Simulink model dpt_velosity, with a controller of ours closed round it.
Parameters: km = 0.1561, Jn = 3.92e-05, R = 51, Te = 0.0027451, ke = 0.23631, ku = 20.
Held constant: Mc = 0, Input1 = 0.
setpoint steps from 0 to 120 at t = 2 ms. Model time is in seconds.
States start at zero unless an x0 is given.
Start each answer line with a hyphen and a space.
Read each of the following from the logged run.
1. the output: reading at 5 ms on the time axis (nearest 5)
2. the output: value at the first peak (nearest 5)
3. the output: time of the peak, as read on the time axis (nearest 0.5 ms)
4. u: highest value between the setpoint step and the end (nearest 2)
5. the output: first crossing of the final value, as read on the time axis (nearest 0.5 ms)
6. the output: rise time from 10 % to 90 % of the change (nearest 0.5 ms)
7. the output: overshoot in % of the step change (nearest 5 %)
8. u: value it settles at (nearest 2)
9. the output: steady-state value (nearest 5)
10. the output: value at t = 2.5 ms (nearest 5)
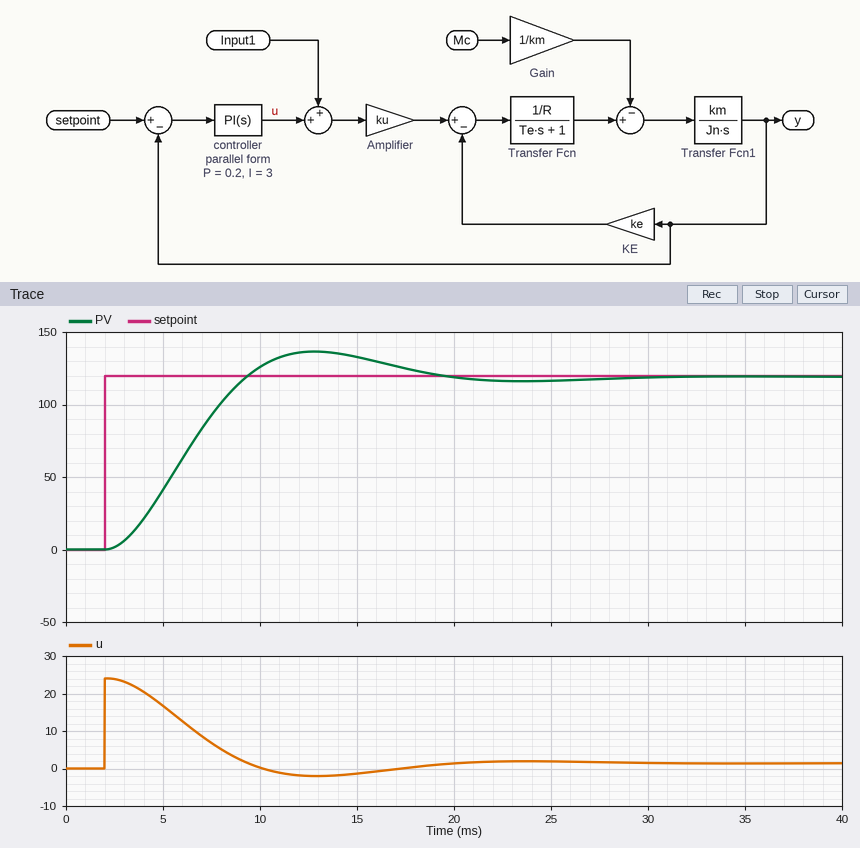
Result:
- 40
- 135
- 13.0 ms
- 24
- 9.5 ms
- 5.0 ms
- 15 %
- 2
- 120
- 0
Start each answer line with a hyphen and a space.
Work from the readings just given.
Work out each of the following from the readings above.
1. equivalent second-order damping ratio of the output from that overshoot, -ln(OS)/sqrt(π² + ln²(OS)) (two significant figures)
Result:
- 0.52
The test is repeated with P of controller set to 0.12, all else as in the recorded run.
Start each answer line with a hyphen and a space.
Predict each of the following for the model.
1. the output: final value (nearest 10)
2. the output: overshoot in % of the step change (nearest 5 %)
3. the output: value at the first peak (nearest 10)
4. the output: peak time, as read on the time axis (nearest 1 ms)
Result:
- 120
- 10 %
- 130
- 18 ms
